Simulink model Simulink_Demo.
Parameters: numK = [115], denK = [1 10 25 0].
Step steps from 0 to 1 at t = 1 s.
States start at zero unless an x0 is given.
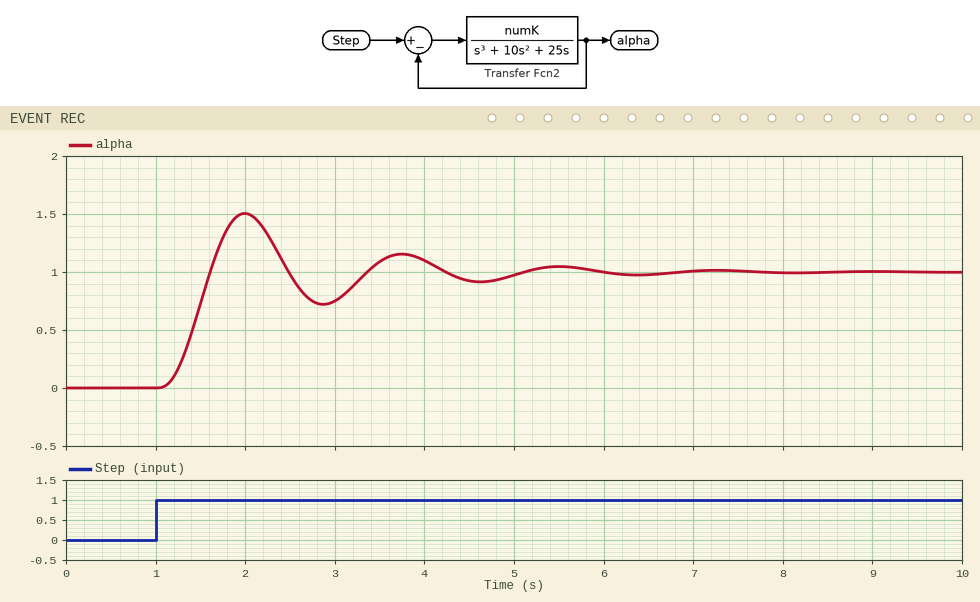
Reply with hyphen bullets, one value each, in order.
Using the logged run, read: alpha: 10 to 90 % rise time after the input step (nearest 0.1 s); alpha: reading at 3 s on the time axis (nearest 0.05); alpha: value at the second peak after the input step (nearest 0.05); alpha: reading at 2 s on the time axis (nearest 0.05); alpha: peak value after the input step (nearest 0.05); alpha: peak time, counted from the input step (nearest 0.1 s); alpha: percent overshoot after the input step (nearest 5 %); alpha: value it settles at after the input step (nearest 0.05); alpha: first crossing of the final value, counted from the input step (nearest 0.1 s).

- 0.4 s
- 0.75
- 1.15
- 1.50
- 1.50
- 1.0 s
- 50 %
- 1.00
- 0.6 s
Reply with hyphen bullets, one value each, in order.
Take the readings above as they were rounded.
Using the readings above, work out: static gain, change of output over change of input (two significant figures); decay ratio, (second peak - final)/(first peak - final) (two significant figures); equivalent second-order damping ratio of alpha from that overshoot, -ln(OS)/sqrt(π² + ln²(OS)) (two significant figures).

- 1.0
- 0.30
- 0.22
